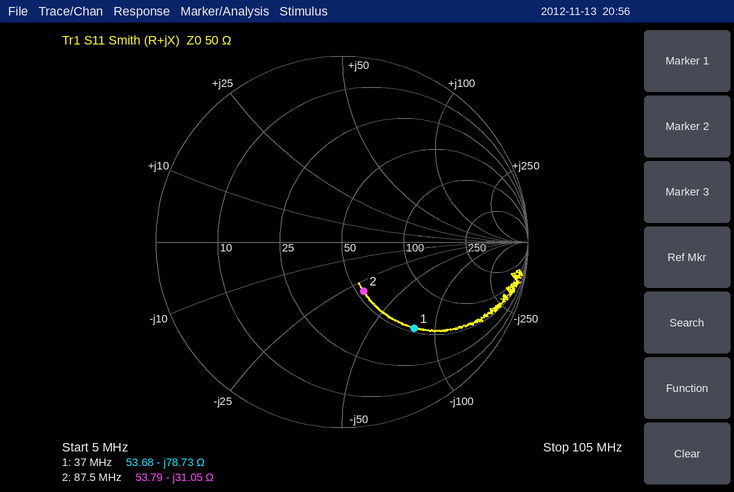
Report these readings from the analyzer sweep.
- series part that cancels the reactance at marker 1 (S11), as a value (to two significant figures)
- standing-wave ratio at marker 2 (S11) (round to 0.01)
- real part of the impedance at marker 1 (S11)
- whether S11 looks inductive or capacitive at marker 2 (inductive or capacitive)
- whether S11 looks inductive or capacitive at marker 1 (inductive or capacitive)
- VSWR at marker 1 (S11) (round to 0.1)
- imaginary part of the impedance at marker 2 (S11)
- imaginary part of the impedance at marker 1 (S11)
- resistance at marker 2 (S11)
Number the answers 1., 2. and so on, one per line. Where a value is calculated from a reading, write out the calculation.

1. L = 78.73 Ω/(2π × 37 MHz) ≈ 339 nH, so 340 nH to two significant figures
2. 1.81
3. 53.68 Ω
4. capacitive
5. capacitive
6. 4.1
7. -31.05 Ω
8. -78.73 Ω
9. 53.79 Ω
